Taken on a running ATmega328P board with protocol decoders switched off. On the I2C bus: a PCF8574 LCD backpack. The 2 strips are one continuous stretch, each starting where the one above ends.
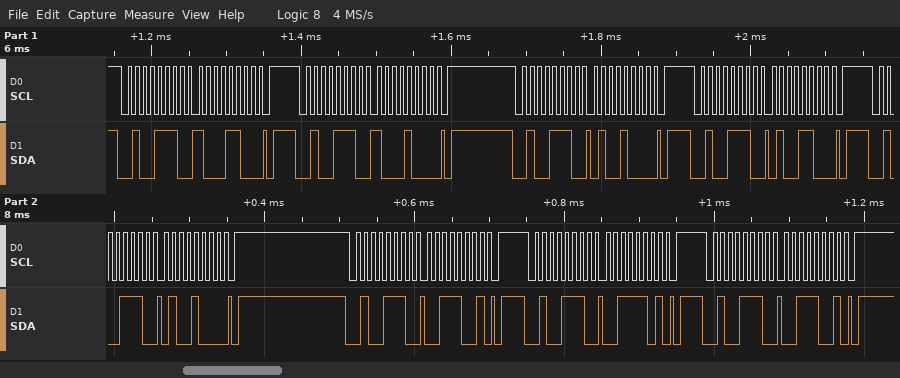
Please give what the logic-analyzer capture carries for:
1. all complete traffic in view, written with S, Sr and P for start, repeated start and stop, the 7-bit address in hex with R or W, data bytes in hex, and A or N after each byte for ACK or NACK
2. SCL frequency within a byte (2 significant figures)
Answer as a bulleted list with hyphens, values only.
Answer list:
- S 27W A 8C A P S 27W A 88 A P S 27W A 48 A P S 27W A 4C A P S 27W A 48 A P S 27W A 39 A P S 27W A 3D A P S 27W A 39 A P
- 100 kHz
